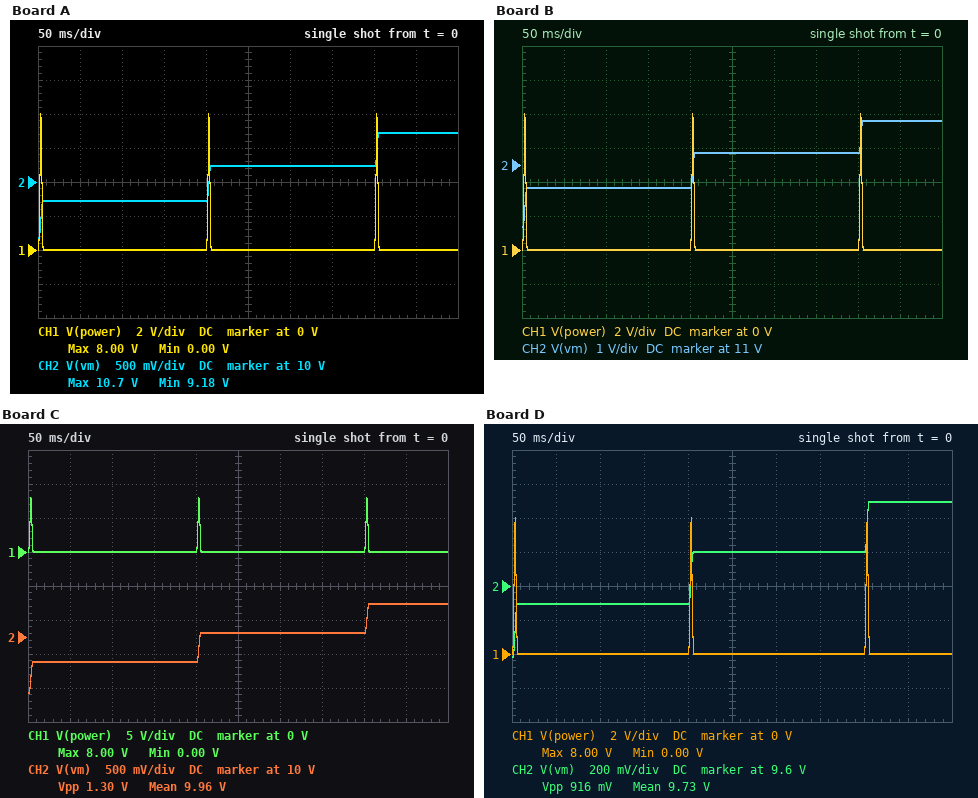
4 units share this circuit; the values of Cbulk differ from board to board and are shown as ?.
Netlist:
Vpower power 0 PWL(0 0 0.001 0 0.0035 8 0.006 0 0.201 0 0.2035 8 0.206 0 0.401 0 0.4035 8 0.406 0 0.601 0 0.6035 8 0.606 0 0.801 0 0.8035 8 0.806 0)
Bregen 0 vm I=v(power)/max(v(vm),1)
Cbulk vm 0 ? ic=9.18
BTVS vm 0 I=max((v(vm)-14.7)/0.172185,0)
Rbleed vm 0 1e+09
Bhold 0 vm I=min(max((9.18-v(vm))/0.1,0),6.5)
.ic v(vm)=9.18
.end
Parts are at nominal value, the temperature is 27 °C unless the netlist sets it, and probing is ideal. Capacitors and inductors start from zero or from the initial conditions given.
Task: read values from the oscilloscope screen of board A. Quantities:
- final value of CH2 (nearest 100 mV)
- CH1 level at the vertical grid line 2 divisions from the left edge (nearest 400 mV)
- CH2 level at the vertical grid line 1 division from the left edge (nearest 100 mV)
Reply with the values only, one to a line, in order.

10.7 V
0 V
9.7 V
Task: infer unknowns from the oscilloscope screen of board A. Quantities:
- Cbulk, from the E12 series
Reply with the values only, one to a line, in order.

3.9 mF
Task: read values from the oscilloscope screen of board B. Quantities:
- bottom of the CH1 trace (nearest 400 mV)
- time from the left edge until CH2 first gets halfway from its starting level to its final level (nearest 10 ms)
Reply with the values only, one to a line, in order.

0 V
200 ms
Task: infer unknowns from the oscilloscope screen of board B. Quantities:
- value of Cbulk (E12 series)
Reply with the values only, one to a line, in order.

1.8 mF
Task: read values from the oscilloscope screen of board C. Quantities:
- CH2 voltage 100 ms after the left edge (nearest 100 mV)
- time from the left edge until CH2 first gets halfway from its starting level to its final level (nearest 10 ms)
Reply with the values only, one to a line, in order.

9.6 V
200 ms
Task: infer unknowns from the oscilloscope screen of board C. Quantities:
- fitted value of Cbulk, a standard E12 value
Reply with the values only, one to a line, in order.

4.7 mF
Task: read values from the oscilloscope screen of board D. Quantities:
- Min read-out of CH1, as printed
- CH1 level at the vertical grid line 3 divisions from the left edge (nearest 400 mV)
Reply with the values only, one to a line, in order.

0.00 V
0 V
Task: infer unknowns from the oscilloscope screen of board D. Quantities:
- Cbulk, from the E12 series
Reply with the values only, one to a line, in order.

6.8 mF
